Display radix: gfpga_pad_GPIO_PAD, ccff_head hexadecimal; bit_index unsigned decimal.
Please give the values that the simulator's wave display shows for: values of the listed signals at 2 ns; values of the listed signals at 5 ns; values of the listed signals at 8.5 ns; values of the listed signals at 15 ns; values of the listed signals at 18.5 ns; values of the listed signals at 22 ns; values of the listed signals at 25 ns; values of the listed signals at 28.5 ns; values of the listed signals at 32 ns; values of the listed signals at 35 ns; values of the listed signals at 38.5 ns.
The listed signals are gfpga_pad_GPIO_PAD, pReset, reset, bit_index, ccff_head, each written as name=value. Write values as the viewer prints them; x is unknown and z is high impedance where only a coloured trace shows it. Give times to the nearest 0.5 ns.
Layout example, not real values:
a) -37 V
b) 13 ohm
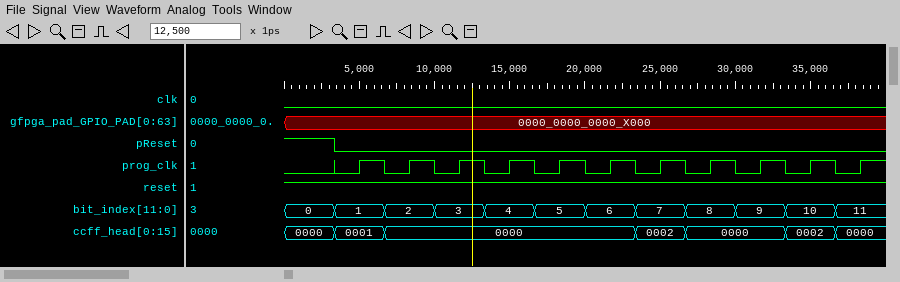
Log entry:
a) gfpga_pad_GPIO_PAD=0000_0000_0000_X000, pReset=1, reset=1, bit_index=0, ccff_head=0000
b) gfpga_pad_GPIO_PAD=0000_0000_0000_X000, pReset=0, reset=1, bit_index=1, ccff_head=0001
c) gfpga_pad_GPIO_PAD=0000_0000_0000_X000, pReset=0, reset=1, bit_index=2, ccff_head=0000
d) gfpga_pad_GPIO_PAD=0000_0000_0000_X000, pReset=0, reset=1, bit_index=4, ccff_head=0000
e) gfpga_pad_GPIO_PAD=0000_0000_0000_X000, pReset=0, reset=1, bit_index=5, ccff_head=0000
f) gfpga_pad_GPIO_PAD=0000_0000_0000_X000, pReset=0, reset=1, bit_index=6, ccff_head=0000
g) gfpga_pad_GPIO_PAD=0000_0000_0000_X000, pReset=0, reset=1, bit_index=7, ccff_head=0002
h) gfpga_pad_GPIO_PAD=0000_0000_0000_X000, pReset=0, reset=1, bit_index=8, ccff_head=0000
i) gfpga_pad_GPIO_PAD=0000_0000_0000_X000, pReset=0, reset=1, bit_index=9, ccff_head=0000
j) gfpga_pad_GPIO_PAD=0000_0000_0000_X000, pReset=0, reset=1, bit_index=10, ccff_head=0002
k) gfpga_pad_GPIO_PAD=0000_0000_0000_X000, pReset=0, reset=1, bit_index=11, ccff_head=0000
